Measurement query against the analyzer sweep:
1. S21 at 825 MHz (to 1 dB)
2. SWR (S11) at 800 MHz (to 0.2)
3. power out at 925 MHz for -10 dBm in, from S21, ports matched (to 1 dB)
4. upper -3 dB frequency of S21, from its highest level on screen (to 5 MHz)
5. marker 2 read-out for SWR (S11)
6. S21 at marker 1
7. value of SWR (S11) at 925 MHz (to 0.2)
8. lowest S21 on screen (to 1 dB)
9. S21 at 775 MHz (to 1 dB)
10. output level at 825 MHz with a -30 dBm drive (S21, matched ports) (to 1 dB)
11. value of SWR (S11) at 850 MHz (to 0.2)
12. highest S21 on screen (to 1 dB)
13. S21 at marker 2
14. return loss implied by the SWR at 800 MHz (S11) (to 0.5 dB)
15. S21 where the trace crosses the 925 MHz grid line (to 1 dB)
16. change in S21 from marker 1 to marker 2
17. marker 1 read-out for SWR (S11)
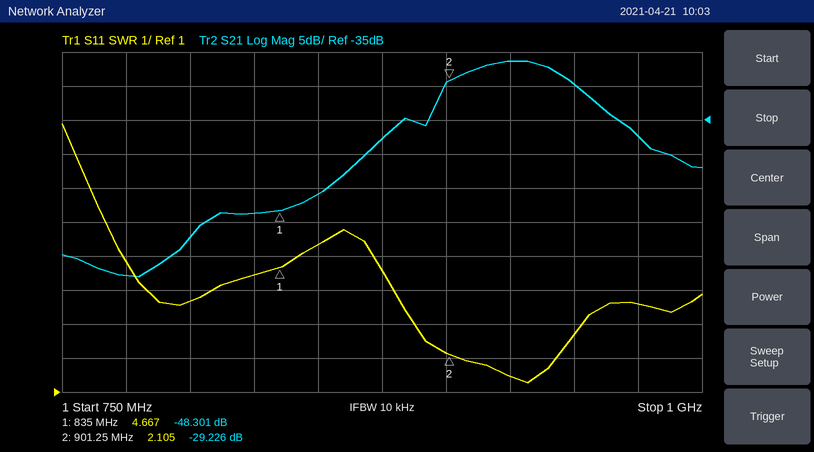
-49 dB
3.6
-36 dBm
950 MHz
2.105
-48.301 dB
1.4
-58 dB
-58 dB
-79 dBm
5.4
-26 dB
-29.226 dB
5.0 dB
-26 dB
19.075 dB
4.667
